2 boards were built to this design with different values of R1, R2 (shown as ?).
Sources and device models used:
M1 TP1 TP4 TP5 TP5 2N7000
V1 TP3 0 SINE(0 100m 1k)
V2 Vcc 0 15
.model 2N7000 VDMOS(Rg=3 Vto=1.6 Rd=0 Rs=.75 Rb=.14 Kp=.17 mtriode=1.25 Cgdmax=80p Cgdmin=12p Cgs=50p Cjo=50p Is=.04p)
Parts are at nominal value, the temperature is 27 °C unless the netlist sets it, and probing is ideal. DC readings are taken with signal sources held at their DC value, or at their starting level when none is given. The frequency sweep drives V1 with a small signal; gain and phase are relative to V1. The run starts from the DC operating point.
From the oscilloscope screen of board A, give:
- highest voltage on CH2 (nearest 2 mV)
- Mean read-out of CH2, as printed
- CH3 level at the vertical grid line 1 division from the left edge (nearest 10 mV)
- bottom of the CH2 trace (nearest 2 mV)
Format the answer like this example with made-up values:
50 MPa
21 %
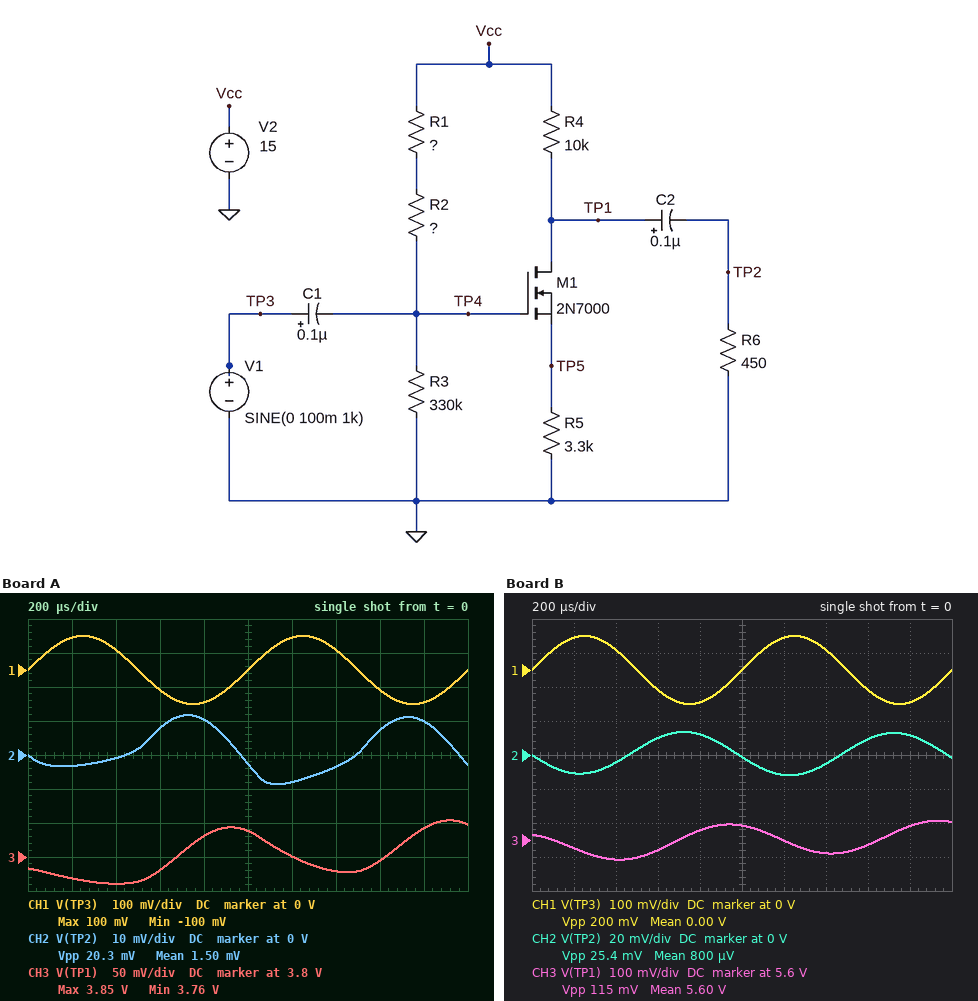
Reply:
12 mV
1.50 mV
3.77 V
-8 mV
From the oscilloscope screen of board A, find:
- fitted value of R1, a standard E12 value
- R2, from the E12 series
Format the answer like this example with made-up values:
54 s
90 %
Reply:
120 kΩ
470 kΩ
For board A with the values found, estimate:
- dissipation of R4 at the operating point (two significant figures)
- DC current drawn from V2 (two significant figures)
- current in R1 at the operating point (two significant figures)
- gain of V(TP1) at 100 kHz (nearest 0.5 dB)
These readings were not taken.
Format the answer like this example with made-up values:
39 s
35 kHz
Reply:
13 mW
1.1 mA
16 µA
-20.0 dB
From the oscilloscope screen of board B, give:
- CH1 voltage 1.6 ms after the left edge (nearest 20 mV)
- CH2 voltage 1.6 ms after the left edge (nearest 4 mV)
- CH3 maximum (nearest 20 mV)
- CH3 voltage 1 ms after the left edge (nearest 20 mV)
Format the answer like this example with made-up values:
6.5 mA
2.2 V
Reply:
-60 mV
8 mV
5.66 V
5.64 V
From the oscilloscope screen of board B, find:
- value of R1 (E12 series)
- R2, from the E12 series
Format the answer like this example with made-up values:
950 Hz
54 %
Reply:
150 kΩ
560 kΩ
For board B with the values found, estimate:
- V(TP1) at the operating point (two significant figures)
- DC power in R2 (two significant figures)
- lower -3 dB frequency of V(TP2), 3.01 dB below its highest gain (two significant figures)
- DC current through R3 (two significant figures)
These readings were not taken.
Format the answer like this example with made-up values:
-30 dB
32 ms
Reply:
5.6 V
120 µW
8.3 MHz
14 µA
